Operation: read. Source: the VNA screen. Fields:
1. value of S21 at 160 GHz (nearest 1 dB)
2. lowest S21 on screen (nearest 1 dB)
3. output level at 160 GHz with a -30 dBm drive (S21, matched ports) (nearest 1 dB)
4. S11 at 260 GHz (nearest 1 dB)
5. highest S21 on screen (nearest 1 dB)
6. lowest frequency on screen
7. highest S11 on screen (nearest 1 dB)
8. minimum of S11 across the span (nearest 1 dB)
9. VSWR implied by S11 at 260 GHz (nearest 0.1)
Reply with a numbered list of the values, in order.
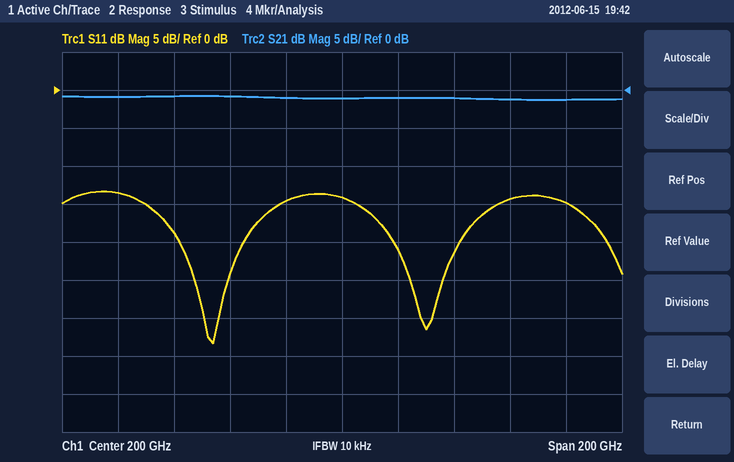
1. -1 dB
2. -1 dB
3. -31 dBm
4. -14 dB
5. -1 dB
6. 100 GHz
7. -13 dB
8. -33 dB
9. 1.5
